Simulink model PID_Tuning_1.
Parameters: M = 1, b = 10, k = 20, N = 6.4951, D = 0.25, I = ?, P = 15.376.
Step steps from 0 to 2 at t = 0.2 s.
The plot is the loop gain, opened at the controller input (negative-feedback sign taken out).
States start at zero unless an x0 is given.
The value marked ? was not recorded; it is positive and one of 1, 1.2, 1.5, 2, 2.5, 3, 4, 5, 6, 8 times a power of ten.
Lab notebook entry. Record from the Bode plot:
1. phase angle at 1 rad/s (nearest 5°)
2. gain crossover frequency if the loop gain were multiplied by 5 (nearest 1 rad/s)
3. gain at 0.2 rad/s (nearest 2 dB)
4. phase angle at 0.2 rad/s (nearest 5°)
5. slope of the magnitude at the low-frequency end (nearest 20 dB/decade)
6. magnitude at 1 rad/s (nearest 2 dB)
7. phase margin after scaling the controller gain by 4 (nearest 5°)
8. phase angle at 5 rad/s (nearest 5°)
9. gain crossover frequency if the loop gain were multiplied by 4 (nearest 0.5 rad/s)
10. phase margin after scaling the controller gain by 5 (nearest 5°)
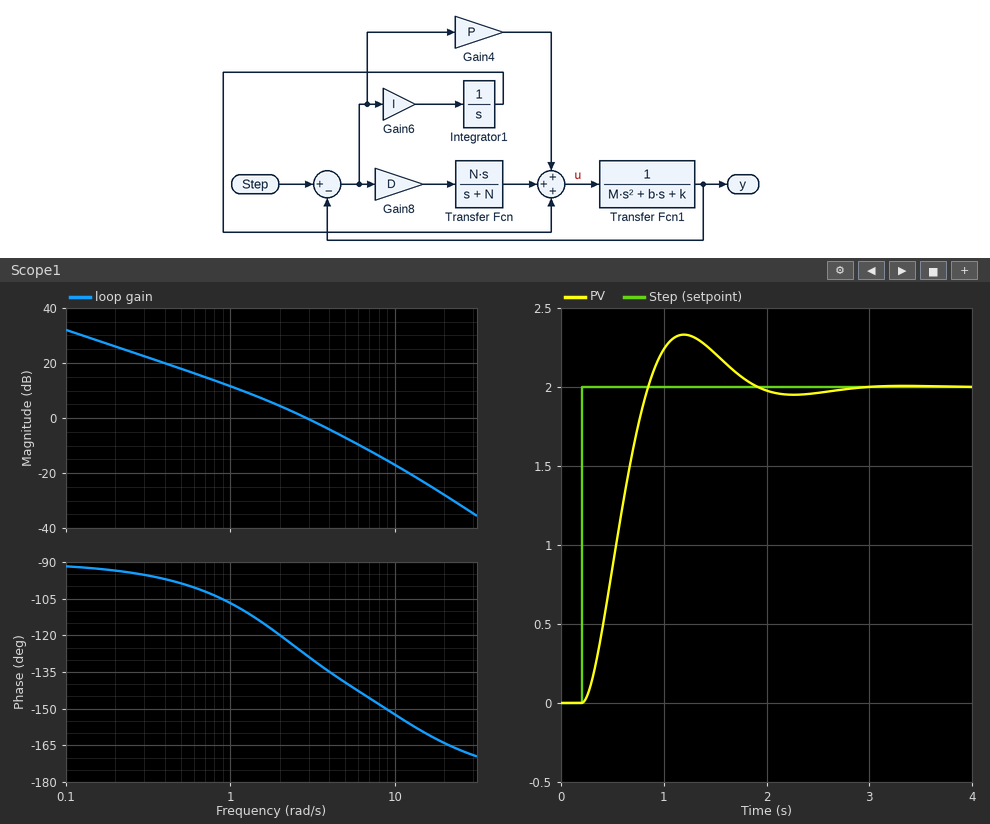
-105°
8 rad/s
26 dB
-95°
-20 dB/decade
12 dB
35°
-140°
7.0 rad/s
30°
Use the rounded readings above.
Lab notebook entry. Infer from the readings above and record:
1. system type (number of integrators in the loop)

1
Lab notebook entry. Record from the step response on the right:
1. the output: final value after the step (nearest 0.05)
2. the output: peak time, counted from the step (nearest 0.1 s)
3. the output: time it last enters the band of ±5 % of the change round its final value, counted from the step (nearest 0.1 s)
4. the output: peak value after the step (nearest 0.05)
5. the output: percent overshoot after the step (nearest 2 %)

2.00
1.0 s
1.5 s
2.35
16 %
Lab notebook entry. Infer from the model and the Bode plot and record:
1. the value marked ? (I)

80
